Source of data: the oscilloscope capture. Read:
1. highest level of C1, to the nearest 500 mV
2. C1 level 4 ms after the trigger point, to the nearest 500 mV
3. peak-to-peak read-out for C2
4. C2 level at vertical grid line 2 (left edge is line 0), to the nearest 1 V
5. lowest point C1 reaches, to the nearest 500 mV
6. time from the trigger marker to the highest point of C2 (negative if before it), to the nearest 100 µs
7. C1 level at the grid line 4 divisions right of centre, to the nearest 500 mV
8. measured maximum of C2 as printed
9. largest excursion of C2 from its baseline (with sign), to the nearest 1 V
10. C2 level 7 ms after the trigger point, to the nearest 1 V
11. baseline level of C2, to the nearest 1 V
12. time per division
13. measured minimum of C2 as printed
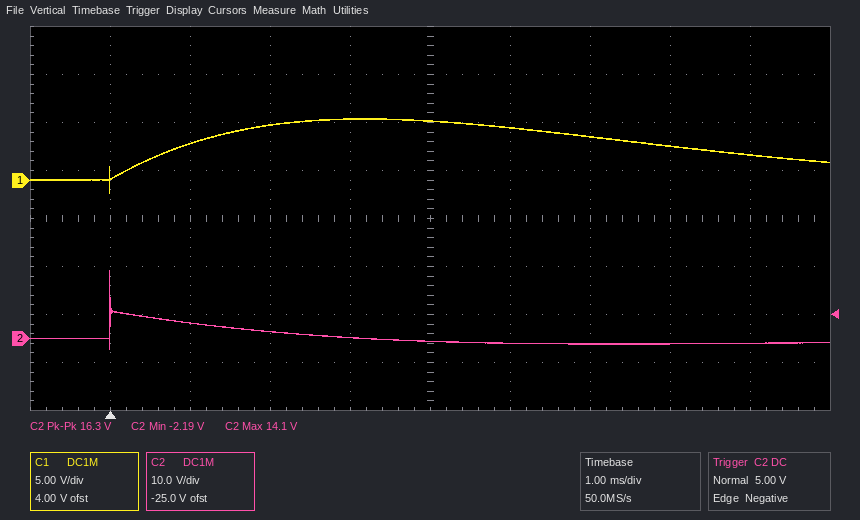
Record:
6.5 V
6.0 V
16.3 V
3 V
-1.5 V
0.0 ms
2.5 V
14.1 V
+15 V
-1 V
-1 V
1 ms
-2.19 V
